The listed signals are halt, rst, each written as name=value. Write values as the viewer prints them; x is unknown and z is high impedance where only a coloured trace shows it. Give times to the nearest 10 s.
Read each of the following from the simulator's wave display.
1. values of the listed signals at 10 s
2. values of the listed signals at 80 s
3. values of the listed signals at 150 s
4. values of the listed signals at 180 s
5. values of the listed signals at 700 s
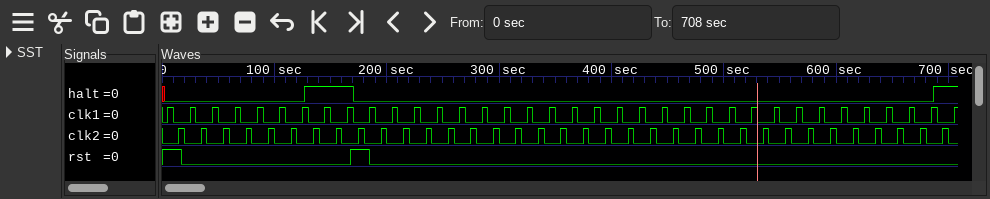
halt=0, rst=1
halt=0, rst=0
halt=1, rst=0
halt=0, rst=1
halt=1, rst=0
